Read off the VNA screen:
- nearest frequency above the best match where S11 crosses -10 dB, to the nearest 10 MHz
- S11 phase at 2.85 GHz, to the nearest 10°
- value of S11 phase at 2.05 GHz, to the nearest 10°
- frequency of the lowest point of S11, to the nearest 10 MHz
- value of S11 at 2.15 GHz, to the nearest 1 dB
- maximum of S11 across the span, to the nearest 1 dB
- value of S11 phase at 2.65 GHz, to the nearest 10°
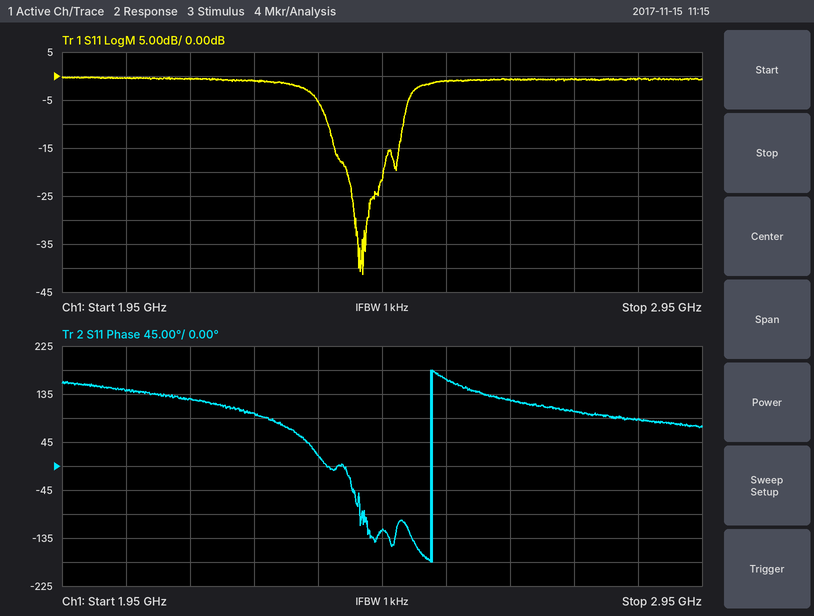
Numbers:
2.48 GHz
90°
140°
2.42 GHz
-1 dB
0 dB
120°
